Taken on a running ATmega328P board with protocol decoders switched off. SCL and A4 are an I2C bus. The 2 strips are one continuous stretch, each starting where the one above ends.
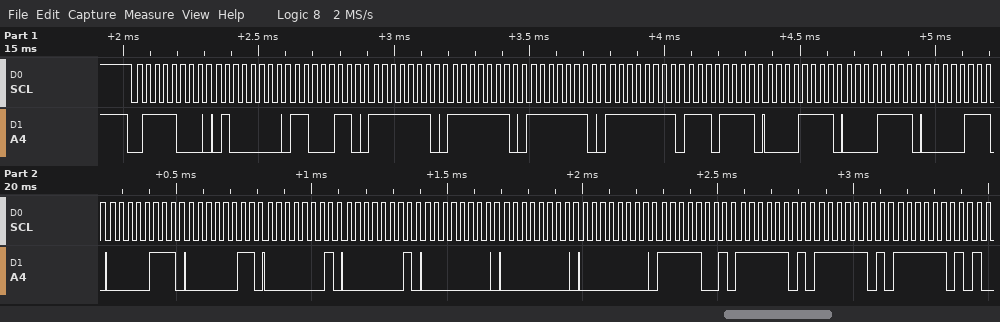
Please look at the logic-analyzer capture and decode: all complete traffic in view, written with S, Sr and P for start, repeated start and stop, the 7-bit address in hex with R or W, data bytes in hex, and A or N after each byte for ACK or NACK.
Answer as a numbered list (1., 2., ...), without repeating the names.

1. S 3CW A 40 A C6 A FE A FE A FE A FF A EF A 0F A 0F A 07 A 07 A 03 A 01 A 01 A 00 A 00 A 00 A F9 A FD A FD A FD A
